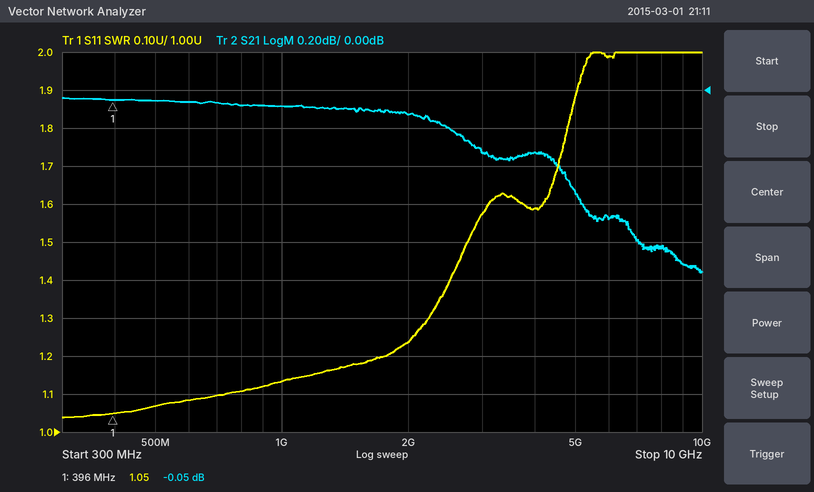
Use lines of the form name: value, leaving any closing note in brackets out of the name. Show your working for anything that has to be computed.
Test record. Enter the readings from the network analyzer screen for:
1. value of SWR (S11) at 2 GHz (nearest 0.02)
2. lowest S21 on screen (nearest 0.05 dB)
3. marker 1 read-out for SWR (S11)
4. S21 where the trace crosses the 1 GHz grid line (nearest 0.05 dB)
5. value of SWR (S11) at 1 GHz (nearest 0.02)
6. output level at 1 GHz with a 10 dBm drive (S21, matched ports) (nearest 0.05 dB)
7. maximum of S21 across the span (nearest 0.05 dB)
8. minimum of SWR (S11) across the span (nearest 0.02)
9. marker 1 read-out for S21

value of SWR (S11) at 2 GHz: 1.24
lowest S21 on screen: -0.95 dB
marker 1 read-out for SWR: 1.05
S21 where the trace crosses the 1 GHz grid line: -0.10 dB
value of SWR (S11) at 1 GHz: 1.14
output level at 1 GHz with a 10 dBm drive (S21, matched ports): 10 dBm + (-0.10 dB) = 9.90 dBm
maximum of S21 across the span: -0.05 dB
minimum of SWR (S11) across the span: 1.04
marker 1 read-out for S21: -0.05 dB
